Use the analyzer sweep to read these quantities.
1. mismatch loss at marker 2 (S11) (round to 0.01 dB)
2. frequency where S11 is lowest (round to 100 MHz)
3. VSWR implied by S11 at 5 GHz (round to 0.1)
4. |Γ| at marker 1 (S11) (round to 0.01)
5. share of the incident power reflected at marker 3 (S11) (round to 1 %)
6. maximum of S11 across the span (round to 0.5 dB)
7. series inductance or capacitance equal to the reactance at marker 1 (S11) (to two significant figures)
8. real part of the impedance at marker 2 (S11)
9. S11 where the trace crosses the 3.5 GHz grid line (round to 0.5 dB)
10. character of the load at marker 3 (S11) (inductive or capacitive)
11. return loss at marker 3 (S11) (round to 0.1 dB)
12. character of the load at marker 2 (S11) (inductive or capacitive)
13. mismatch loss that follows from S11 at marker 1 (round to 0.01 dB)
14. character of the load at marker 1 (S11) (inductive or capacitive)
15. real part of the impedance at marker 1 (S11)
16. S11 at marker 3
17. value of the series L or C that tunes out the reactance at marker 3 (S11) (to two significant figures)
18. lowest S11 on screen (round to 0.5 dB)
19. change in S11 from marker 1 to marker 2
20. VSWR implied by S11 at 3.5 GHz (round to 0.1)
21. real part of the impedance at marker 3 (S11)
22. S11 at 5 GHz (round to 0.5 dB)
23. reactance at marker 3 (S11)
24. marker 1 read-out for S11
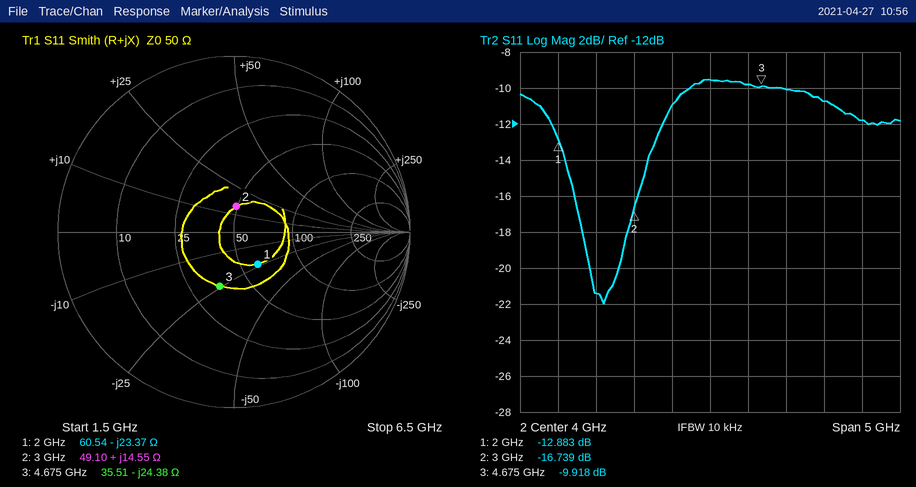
0.09 dB
2.6 GHz
1.9
0.23
10 %
-9.5 dB
3.4 pF
49.10 Ω
-11.0 dB
capacitive
9.9 dB
inductive
0.23 dB
capacitive
60.54 Ω
-9.918 dB
830 pH
-22.0 dB
-3.856 dB
1.8
35.51 Ω
-10.0 dB
-24.38 Ω
-12.883 dB
